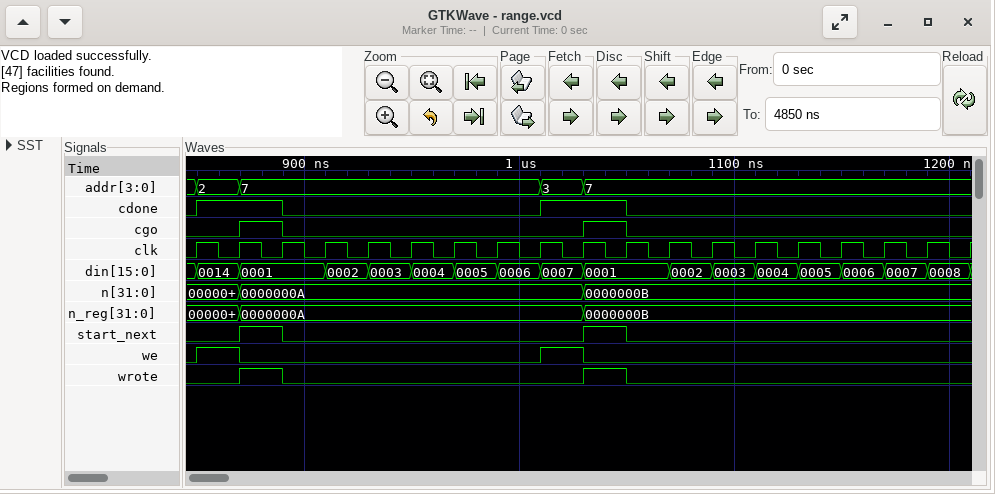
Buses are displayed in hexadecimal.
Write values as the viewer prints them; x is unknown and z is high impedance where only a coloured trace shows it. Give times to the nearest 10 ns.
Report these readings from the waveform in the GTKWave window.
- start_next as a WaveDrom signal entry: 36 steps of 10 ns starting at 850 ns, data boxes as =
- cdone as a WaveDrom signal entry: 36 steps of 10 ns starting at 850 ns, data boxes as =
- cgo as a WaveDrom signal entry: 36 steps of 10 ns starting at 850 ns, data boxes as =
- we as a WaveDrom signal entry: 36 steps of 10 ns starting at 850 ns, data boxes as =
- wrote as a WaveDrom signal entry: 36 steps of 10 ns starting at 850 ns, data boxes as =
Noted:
{name: 'start_next', wave: '0.1.0.............1.0...............'}
{name: 'cdone', wave: '1...0...........1...0...............'}
{name: 'cgo', wave: '0.1.0.............1.0...............'}
{name: 'we', wave: '1.0.............1.0.................'}
{name: 'wrote', wave: '0.1.0.............1.0...............'}
